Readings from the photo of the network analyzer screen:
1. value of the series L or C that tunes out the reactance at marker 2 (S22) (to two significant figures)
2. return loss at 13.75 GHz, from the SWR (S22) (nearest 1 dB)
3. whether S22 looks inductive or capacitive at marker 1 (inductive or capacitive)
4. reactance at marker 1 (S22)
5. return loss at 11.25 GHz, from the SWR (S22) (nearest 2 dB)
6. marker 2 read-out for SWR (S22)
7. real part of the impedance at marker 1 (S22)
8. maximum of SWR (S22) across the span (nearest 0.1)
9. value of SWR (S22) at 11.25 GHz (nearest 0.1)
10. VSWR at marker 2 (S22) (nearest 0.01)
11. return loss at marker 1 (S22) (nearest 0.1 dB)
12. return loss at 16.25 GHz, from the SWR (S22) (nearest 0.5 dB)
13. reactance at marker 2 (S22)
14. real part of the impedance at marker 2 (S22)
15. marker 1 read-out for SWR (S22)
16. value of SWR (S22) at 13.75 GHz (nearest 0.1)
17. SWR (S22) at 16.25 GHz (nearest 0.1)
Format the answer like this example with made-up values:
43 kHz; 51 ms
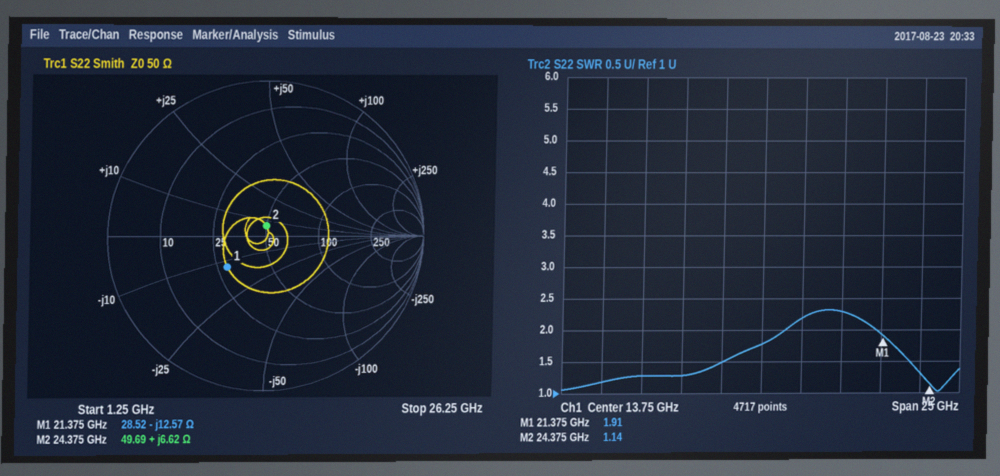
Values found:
990 fF; 11 dB; capacitive; -12.57 Ω; 14 dB; 1.14; 28.52 Ω; 2.3; 1.5; 1.14; 10.1 dB; 8.5 dB; +6.62 Ω; 49.69 Ω; 1.91; 1.8; 2.2
